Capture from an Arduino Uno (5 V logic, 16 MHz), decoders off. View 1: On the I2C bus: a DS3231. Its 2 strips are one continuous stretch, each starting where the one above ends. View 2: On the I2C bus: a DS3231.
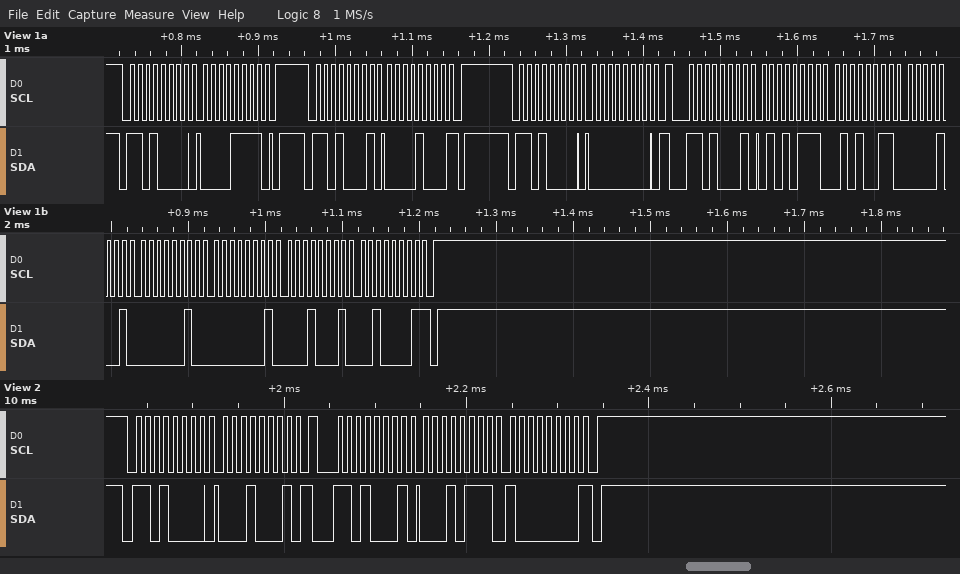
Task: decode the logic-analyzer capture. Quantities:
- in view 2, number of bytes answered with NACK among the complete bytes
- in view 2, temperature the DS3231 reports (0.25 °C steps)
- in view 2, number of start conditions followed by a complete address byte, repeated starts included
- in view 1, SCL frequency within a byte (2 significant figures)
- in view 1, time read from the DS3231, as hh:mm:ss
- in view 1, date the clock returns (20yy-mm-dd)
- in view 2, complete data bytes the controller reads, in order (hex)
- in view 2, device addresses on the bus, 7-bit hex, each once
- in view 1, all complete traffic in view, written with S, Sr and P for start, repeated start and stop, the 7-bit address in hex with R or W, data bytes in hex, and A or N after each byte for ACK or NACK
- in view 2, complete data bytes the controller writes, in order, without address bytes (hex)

1
23.50 °C
2
100 kHz
09:53:57
2021-11-01
17 80
0x68
S 68W A 0F A P S 68R A 08 N P S 68W A 00 A Sr 68R A 57 A 53 A 09 A 02 A 01 A 11 A 21 N P
11
